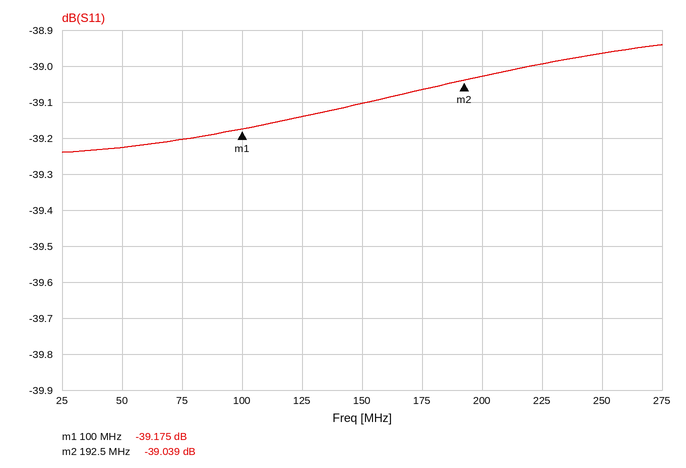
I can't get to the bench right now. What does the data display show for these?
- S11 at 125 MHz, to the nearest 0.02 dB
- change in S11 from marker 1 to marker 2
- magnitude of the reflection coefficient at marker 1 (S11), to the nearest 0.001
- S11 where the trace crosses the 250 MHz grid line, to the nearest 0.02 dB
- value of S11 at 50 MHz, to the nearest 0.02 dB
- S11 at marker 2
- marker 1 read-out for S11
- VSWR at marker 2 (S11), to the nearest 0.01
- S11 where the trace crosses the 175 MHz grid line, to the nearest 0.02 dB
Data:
-39.14 dB
0.136 dB
0.011
-38.96 dB
-39.22 dB
-39.039 dB
-39.175 dB
1.02
-39.06 dB
